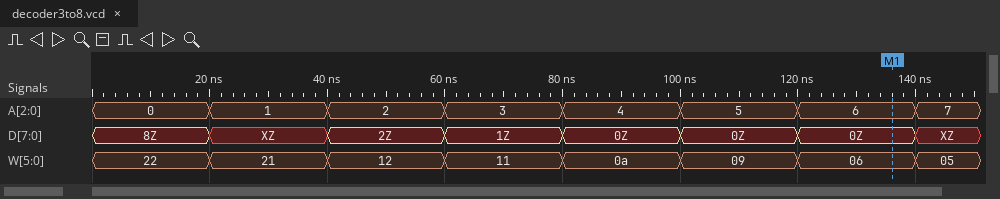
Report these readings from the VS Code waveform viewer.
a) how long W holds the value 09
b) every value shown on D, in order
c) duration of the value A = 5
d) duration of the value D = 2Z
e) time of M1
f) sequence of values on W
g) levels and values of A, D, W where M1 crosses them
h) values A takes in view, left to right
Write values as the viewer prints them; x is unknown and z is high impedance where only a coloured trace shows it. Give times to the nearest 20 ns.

20 ns
8Z, XZ, 2Z, 1Z, 0Z, 0Z, 0Z, XZ
20 ns
20 ns
140 ns
22, 21, 12, 11, 0a, 09, 06, 05
A=6, D=0Z, W=06
0, 1, 2, 3, 4, 5, 6, 7
